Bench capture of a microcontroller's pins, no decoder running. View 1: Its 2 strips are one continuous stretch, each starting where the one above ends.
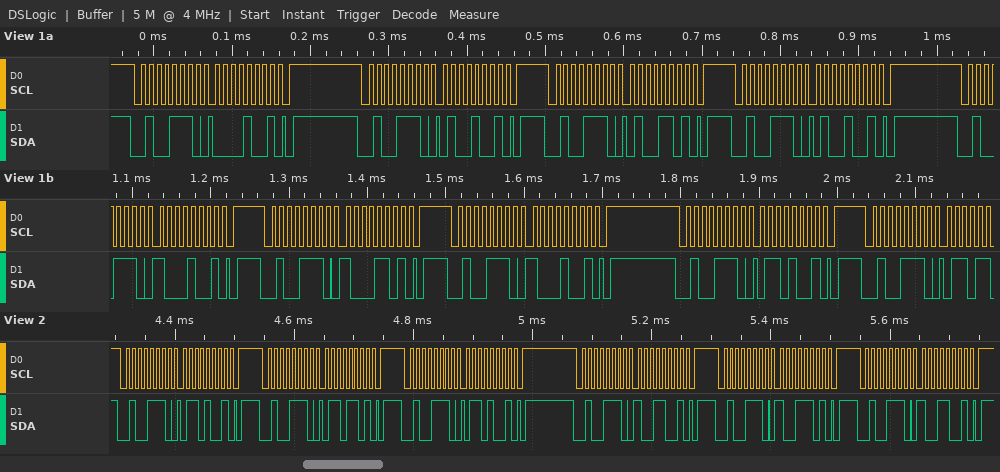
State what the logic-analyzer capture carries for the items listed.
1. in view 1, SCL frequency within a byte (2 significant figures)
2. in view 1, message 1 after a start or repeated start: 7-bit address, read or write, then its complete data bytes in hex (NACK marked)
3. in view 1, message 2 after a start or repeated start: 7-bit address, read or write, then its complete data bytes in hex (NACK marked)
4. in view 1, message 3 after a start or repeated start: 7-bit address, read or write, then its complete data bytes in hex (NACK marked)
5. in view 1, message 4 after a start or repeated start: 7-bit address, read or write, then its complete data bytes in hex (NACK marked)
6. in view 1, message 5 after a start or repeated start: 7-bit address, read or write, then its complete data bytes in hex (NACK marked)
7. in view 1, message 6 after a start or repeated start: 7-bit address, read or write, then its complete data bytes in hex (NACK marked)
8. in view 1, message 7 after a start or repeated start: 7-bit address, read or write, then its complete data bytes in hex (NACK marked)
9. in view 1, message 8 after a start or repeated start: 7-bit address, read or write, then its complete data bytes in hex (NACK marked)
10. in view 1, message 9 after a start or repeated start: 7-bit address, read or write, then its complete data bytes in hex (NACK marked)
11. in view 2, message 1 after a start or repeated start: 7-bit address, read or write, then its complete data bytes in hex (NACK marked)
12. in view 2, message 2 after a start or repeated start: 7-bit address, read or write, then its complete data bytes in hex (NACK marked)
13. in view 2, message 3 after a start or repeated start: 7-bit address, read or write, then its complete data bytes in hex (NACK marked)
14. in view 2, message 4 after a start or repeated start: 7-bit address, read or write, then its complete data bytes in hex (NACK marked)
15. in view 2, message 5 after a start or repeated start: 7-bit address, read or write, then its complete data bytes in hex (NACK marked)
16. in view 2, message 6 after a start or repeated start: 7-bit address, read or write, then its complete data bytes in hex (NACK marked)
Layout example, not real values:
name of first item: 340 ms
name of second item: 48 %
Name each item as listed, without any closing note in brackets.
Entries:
in view 1, SCL frequency within a byte: 100 kHz
in view 1, message 1 after a start or repeated start: 7-bit address, read or write, then its complete data bytes in hex: 0x27 write: 09
in view 1, message 2 after a start or repeated start: 7-bit address, read or write, then its complete data bytes in hex: 0x27 write: 49
in view 1, message 3 after a start or repeated start: 7-bit address, read or write, then its complete data bytes in hex: 0x27 write: 4D
in view 1, message 4 after a start or repeated start: 7-bit address, read or write, then its complete data bytes in hex: 0x27 write: 49
in view 1, message 5 after a start or repeated start: 7-bit address, read or write, then its complete data bytes in hex: 0x27 write: 89
in view 1, message 6 after a start or repeated start: 7-bit address, read or write, then its complete data bytes in hex: 0x27 write: 8D
in view 1, message 7 after a start or repeated start: 7-bit address, read or write, then its complete data bytes in hex: 0x27 write: 89
in view 1, message 8 after a start or repeated start: 7-bit address, read or write, then its complete data bytes in hex: 0x27 write: 69
in view 1, message 9 after a start or repeated start: 7-bit address, read or write, then its complete data bytes in hex: 0x27 write
in view 2, message 1 after a start or repeated start: 7-bit address, read or write, then its complete data bytes in hex: 0x27 write: 69
in view 2, message 2 after a start or repeated start: 7-bit address, read or write, then its complete data bytes in hex: 0x27 write: 6D
in view 2, message 3 after a start or repeated start: 7-bit address, read or write, then its complete data bytes in hex: 0x27 write: 69
in view 2, message 4 after a start or repeated start: 7-bit address, read or write, then its complete data bytes in hex: 0x27 write: 99
in view 2, message 5 after a start or repeated start: 7-bit address, read or write, then its complete data bytes in hex: 0x27 write: 9D
in view 2, message 6 after a start or repeated start: 7-bit address, read or write, then its complete data bytes in hex: 0x27 write: 99
